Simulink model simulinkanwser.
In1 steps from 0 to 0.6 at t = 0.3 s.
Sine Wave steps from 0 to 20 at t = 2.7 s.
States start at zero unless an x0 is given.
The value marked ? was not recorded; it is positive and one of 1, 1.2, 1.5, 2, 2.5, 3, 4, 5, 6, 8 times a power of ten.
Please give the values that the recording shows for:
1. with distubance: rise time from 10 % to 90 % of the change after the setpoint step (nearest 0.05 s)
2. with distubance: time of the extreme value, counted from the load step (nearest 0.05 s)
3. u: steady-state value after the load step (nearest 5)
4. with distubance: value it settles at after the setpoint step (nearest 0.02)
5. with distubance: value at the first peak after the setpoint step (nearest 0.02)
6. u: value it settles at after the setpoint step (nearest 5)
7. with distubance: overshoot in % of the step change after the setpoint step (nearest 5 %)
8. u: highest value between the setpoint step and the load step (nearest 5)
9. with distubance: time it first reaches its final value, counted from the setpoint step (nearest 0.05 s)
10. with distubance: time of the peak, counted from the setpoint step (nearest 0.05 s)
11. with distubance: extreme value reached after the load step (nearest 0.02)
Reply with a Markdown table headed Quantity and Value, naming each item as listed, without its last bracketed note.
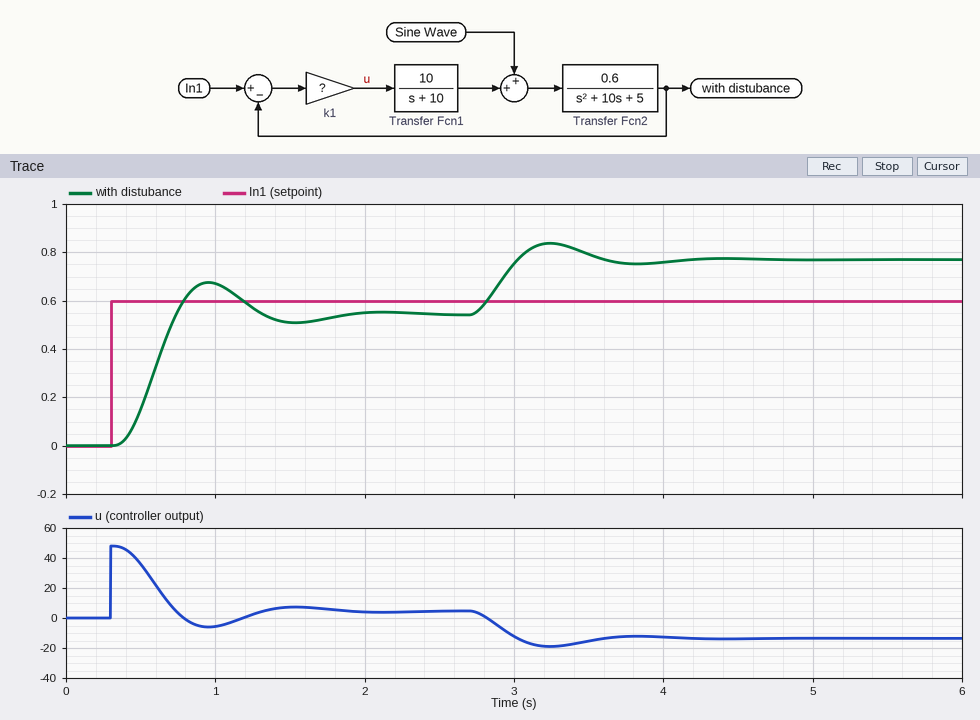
| Quantity | Value |
|---|---|
| with distubance: rise time from 10 % to 90 % of the change after the setpoint step | 0.25 s |
| with distubance: time of the extreme value, counted from the load step | 0.55 s |
| u: steady-state value after the load step | -15 |
| with distubance: value it settles at after the setpoint step | 0.54 |
| with distubance: value at the first peak after the setpoint step | 0.68 |
| u: value it settles at after the setpoint step | 5 |
| with distubance: overshoot in % of the step change after the setpoint step | 25 % |
| u: highest value between the setpoint step and the load step | 50 |
| with distubance: time it first reaches its final value, counted from the setpoint step | 0.45 s |
| with distubance: time of the peak, counted from the setpoint step | 0.65 s |
| with distubance: extreme value reached after the load step | 0.84 |
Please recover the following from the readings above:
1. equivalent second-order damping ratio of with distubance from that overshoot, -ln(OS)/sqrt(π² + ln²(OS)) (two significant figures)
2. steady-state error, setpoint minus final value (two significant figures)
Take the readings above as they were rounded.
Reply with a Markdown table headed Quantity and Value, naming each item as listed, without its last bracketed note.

| Quantity | Value |
|---|---|
| equivalent second-order damping ratio of with distubance from that overshoot, -ln(OS)/sqrt(π² + ln²(OS)) | 0.40 |
| steady-state error, setpoint minus final value | 0.060 |
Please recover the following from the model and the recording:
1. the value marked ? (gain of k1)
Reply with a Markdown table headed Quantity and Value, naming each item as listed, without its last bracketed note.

| Quantity | Value |
|---|---|
| the value marked ? | 80 |
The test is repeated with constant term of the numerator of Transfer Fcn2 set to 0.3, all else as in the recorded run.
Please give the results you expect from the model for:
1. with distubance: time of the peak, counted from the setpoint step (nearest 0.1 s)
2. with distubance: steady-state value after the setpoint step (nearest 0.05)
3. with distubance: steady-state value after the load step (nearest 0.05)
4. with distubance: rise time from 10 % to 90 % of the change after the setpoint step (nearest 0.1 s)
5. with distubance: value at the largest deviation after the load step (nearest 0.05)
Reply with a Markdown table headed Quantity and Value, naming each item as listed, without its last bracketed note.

| Quantity | Value |
|---|---|
| with distubance: time of the peak, counted from the setpoint step | 1.0 s |
| with distubance: steady-state value after the setpoint step | 0.50 |
| with distubance: steady-state value after the load step | 0.70 |
| with distubance: rise time from 10 % to 90 % of the change after the setpoint step | 0.5 s |
| with distubance: value at the largest deviation after the load step | 0.70 |
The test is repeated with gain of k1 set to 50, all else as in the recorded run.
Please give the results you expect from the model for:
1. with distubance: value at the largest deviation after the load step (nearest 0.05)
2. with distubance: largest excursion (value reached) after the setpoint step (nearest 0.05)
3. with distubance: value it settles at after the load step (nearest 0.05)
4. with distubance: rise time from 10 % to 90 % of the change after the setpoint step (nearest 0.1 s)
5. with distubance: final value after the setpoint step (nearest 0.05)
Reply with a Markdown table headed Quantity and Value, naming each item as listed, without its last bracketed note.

| Quantity | Value |
|---|---|
| with distubance: value at the largest deviation after the load step | 0.90 |
| with distubance: largest excursion (value reached) after the setpoint step | 0.55 |
| with distubance: value it settles at after the load step | 0.85 |
| with distubance: rise time from 10 % to 90 % of the change after the setpoint step | 0.4 s |
| with distubance: final value after the setpoint step | 0.50 |
